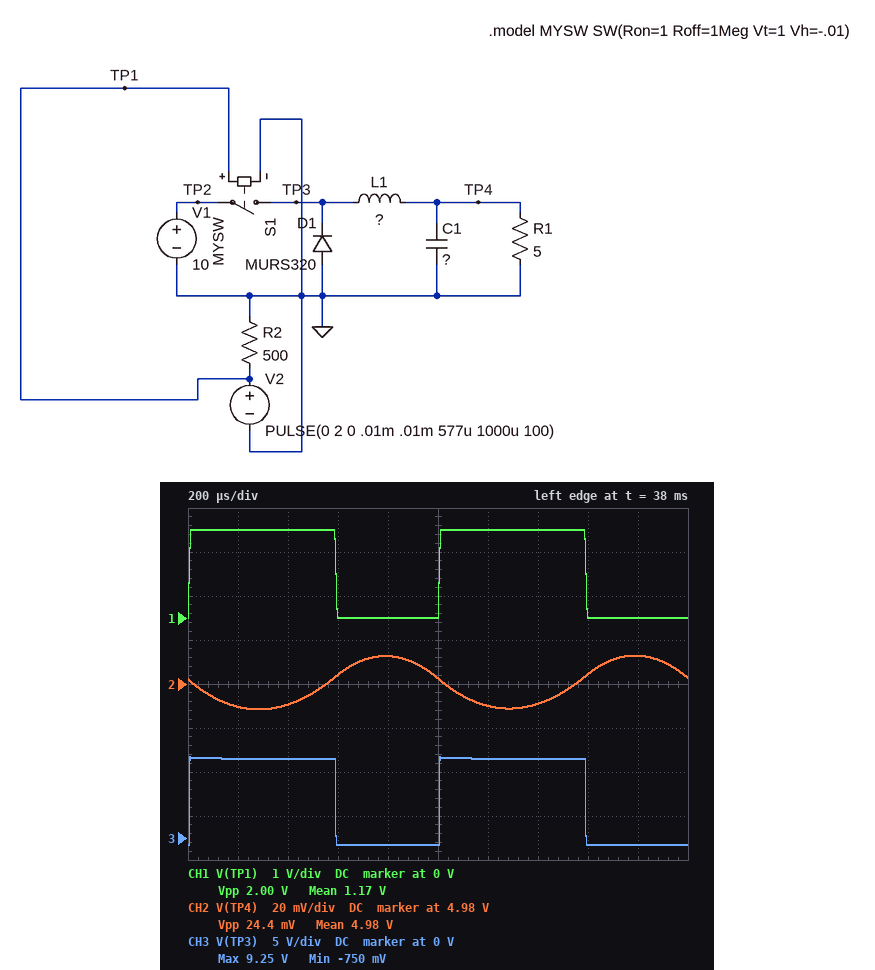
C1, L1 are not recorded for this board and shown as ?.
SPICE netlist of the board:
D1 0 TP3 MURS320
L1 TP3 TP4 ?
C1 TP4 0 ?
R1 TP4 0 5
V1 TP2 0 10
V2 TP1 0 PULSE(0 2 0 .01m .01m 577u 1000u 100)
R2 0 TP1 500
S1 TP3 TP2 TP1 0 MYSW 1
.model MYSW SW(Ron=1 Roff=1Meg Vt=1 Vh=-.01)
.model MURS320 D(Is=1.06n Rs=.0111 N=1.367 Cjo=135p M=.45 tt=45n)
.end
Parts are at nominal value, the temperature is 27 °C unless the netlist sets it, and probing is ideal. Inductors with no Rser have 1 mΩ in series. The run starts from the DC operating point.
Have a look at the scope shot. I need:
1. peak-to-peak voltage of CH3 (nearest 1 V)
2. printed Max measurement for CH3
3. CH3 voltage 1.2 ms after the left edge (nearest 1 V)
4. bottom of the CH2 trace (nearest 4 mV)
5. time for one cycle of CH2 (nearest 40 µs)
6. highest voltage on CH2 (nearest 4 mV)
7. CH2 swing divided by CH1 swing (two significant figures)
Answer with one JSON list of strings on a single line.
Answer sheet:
["10 V", "9.25 V", "9 V", "4.968 V", "1.00 ms", "4.992 V", "0.012"]
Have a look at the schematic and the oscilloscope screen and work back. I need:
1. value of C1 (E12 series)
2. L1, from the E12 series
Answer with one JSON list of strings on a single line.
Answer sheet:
["560 µF", "22 mH"]
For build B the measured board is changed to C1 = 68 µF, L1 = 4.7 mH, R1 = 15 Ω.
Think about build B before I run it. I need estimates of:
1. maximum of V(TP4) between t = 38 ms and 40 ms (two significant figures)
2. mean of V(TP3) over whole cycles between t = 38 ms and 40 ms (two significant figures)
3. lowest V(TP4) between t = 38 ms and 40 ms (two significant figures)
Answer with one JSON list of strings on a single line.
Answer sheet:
["5.9 V", "5.4 V", "4.9 V"]
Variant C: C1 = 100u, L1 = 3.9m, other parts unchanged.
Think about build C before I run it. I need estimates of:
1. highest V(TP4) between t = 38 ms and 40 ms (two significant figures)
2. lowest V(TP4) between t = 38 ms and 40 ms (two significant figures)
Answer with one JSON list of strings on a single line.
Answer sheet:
["5.4 V", "4.6 V"]
